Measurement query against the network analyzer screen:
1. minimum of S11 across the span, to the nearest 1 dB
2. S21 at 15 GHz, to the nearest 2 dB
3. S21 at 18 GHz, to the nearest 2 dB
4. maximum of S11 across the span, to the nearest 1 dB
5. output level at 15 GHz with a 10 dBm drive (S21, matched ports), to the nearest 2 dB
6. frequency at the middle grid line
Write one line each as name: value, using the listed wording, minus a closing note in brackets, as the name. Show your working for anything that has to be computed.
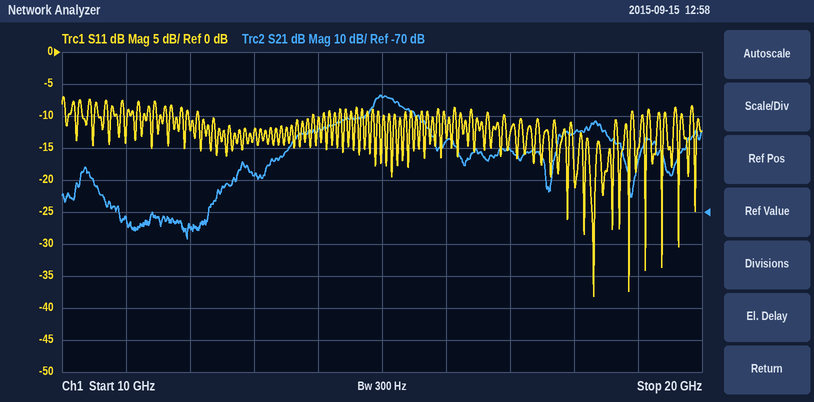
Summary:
minimum of S11 across the span, to the nearest 1 dB: -38 dB
S21 at 15 GHz, to the nearest 2 dB: -34 dB
S21 at 18 GHz, to the nearest 2 dB: -46 dB
maximum of S11 across the span, to the nearest 1 dB: -7 dB
output level at 15 GHz with a 10 dBm drive (S21, matched ports), to the nearest 2 dB: 10 dBm + (-34 dB) = -24 dBm
frequency at the middle grid line: 15 GHz
